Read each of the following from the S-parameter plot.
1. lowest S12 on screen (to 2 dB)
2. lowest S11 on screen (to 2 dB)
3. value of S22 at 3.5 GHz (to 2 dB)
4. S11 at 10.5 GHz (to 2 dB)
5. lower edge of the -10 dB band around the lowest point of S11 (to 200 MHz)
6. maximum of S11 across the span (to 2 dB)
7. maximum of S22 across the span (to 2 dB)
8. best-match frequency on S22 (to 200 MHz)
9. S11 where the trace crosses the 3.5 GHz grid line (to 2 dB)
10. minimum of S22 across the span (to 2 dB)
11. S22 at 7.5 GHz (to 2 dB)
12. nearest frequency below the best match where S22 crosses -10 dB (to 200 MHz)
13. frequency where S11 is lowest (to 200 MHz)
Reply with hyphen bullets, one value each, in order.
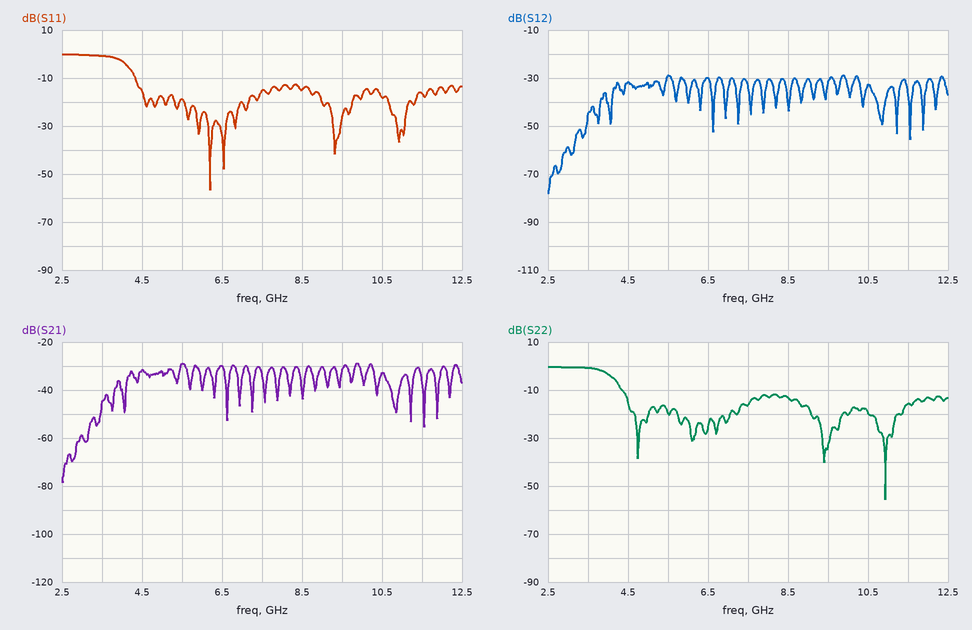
- -78 dB
- -56 dB
- 0 dB
- -18 dB
- 4.4 GHz
- 0 dB
- 0 dB
- 11.0 GHz
- 0 dB
- -56 dB
- -16 dB
- 4.4 GHz
- 6.2 GHz
